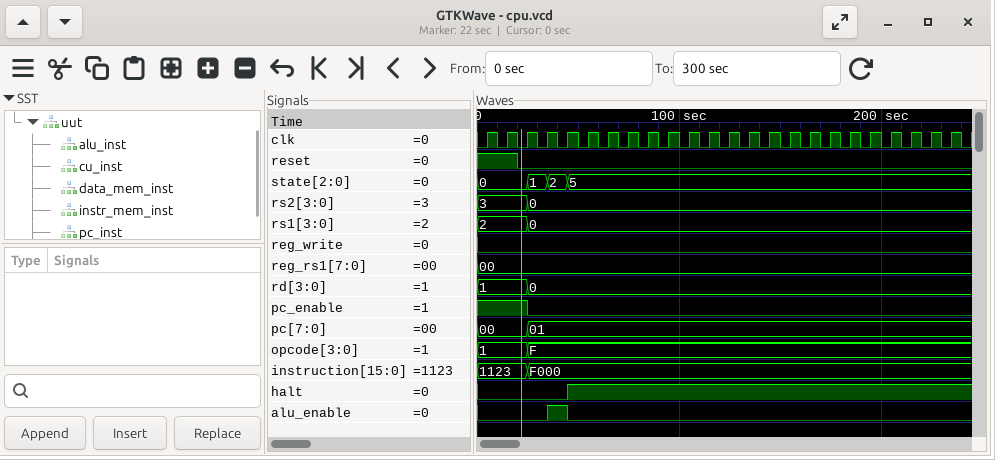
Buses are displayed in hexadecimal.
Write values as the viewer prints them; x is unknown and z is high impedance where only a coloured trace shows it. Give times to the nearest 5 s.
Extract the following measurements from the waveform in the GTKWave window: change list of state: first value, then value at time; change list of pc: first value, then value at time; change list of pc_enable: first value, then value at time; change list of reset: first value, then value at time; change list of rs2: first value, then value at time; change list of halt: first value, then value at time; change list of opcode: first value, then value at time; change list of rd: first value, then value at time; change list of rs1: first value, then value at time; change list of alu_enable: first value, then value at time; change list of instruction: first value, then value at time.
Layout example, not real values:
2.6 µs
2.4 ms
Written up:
0, 1 at 25 s, 2 at 35 s, 5 at 45 s
00, 01 at 25 s
1, 0 at 25 s
1, 0 at 20 s
3, 0 at 25 s
0, 1 at 45 s
1, F at 25 s
1, 0 at 25 s
2, 0 at 25 s
0, 1 at 35 s, 0 at 45 s
1123, F000 at 25 s
